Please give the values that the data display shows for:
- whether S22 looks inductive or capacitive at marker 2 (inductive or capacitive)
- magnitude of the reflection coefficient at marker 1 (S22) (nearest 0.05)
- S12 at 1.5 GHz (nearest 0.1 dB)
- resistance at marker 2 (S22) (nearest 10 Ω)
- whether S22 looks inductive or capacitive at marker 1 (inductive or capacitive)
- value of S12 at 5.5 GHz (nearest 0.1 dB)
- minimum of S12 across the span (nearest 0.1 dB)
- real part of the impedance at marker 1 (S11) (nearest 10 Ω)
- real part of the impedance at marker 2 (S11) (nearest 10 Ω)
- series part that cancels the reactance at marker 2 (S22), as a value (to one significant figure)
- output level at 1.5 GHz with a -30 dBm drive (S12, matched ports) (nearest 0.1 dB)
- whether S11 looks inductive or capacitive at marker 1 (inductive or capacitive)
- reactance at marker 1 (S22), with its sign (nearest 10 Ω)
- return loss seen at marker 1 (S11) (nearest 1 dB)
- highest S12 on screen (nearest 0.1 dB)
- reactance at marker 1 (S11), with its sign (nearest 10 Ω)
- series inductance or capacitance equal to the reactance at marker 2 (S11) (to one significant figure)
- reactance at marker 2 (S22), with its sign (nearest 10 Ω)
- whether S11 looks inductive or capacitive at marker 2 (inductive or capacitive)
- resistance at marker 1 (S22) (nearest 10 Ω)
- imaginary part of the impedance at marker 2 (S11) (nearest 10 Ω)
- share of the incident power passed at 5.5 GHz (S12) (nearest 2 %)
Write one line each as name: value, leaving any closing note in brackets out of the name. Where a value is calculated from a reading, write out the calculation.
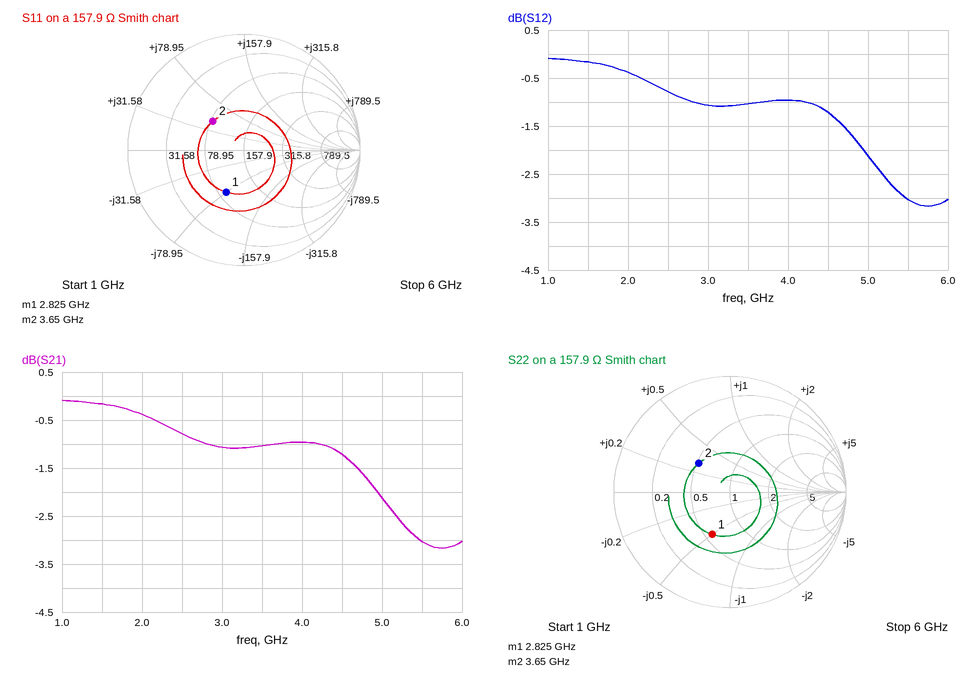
whether S22 looks inductive or capacitive at marker 2: inductive
magnitude of the reflection coefficient at marker 1 (S22): 0.40
S12 at 1.5 GHz: -0.2 dB
resistance at marker 2 (S22): 80 Ω
whether S22 looks inductive or capacitive at marker 1: capacitive
value of S12 at 5.5 GHz: -3.0 dB
minimum of S12 across the span: -3.2 dB
real part of the impedance at marker 1 (S11): 90 Ω
real part of the impedance at marker 2 (S11): 80 Ω
series part that cancels the reactance at marker 2 (S22), as a value: C = 1/(2π × 3.65 GHz × 50 Ω) ≈ 872 fF, so 900 fF to one significant figure
output level at 1.5 GHz with a -30 dBm drive (S12, matched ports): -30 dBm + (-0.2 dB) = -30.2 dBm
whether S11 looks inductive or capacitive at marker 1: capacitive
reactance at marker 1 (S22), with its sign: -80 Ω
return loss seen at marker 1 (S11): 8 dB
highest S12 on screen: -0.1 dB
reactance at marker 1 (S11), with its sign: -80 Ω
series inductance or capacitance equal to the reactance at marker 2 (S11): L = 50 Ω/(2π × 3.65 GHz) ≈ 2 nH
reactance at marker 2 (S22), with its sign: +50 Ω
whether S11 looks inductive or capacitive at marker 2: inductive
resistance at marker 1 (S22): 90 Ω
imaginary part of the impedance at marker 2 (S11): +50 Ω
share of the incident power passed at 5.5 GHz (S12): 10^(-3/10) ≈ 50 %
